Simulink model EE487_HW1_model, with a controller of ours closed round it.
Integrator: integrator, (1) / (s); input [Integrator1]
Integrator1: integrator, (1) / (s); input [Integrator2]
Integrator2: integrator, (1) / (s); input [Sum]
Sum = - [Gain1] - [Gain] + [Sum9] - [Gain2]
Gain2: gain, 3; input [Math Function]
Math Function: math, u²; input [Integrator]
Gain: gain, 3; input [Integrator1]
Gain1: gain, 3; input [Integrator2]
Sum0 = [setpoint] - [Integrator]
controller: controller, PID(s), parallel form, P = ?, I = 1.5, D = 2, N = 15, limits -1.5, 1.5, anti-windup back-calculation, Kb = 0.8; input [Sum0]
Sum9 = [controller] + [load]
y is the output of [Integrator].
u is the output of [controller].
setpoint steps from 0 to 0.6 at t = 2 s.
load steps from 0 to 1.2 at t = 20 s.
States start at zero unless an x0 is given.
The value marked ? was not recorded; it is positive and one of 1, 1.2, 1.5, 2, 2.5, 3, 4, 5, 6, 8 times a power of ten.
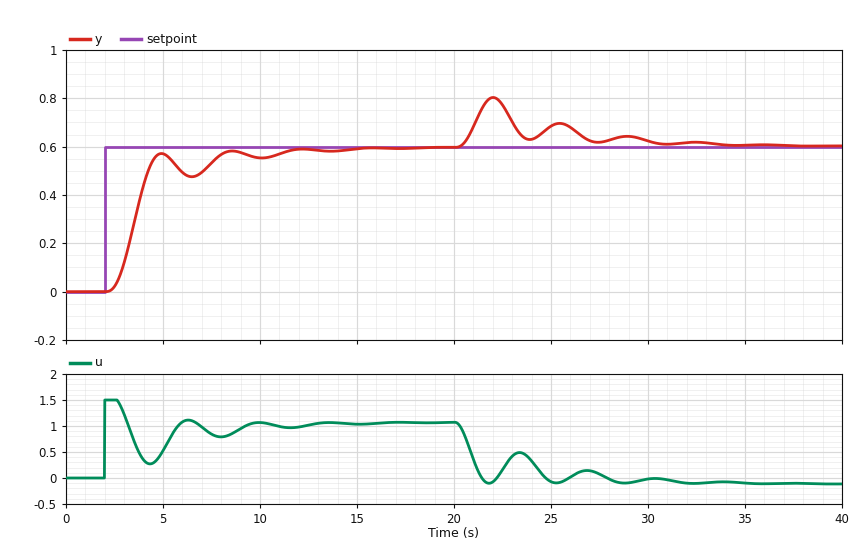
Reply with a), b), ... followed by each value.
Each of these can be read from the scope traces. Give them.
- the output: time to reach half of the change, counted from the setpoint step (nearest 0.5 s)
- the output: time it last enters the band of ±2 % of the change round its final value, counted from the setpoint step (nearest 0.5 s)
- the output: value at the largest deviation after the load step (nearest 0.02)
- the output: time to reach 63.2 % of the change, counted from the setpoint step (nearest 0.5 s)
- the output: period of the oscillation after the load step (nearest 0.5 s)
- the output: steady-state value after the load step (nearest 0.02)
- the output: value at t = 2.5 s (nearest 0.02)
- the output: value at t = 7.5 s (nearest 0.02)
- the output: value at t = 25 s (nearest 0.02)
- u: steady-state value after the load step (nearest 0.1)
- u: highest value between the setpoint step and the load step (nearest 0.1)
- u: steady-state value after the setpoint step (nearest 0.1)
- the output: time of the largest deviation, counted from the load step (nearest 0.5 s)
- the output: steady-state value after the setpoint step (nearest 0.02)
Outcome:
a) 1.5 s
b) 12.5 s
c) 0.80
d) 2.0 s
e) 3.5 s
f) 0.60
g) 0.02
h) 0.54
i) 0.68
j) -0.1
k) 1.5
l) 1.1
m) 2.0 s
n) 0.60
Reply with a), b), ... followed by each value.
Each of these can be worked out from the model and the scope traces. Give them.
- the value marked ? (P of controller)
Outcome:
a) 4
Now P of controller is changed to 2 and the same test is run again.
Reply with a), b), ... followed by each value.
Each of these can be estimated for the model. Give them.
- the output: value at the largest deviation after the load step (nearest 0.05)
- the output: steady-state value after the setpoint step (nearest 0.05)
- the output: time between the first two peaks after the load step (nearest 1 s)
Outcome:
a) 0.85
b) 0.60
c) 4 s
